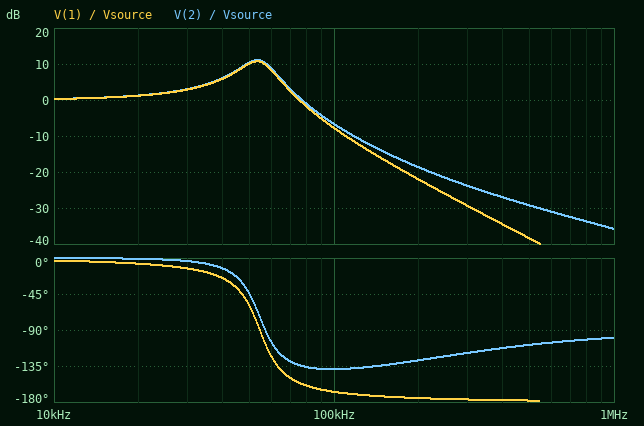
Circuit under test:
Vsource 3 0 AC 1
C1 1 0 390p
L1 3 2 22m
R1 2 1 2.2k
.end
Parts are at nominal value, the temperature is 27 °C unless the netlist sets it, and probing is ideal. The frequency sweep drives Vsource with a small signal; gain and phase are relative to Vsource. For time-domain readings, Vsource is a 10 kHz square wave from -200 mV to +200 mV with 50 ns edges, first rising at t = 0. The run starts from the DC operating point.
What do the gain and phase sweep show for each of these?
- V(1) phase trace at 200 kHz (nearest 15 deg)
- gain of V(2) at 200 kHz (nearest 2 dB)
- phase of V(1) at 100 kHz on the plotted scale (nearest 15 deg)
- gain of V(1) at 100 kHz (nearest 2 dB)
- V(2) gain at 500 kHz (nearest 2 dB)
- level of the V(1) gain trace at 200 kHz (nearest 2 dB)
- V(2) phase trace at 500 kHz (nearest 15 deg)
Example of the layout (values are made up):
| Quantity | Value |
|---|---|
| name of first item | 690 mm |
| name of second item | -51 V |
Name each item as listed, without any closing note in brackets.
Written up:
| Quantity | Value |
|---|---|
| V(1) phase trace at 200 kHz | -180 deg |
| gain of V(2) at 200 kHz | -18 dB |
| phase of V(1) at 100 kHz on the plotted scale | -165 deg |
| gain of V(1) at 100 kHz | -8 dB |
| V(2) gain at 500 kHz | -30 dB |
| level of the V(1) gain trace at 200 kHz | -22 dB |
| V(2) phase trace at 500 kHz | -105 deg |
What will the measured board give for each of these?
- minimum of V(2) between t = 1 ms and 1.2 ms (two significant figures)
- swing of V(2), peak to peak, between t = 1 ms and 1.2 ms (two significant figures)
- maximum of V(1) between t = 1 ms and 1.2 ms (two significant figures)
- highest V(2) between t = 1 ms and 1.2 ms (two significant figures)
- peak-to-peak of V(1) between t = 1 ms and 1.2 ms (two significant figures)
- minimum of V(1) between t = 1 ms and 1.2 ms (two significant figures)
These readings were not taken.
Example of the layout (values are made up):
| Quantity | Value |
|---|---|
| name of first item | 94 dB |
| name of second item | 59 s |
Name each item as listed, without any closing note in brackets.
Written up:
| Quantity | Value |
|---|---|
| minimum of V(2) between t = 1 ms and 1.2 ms | -470 mV |
| swing of V(2), peak to peak, between t = 1 ms and 1.2 ms | 950 mV |
| maximum of V(1) between t = 1 ms and 1.2 ms | 460 mV |
| highest V(2) between t = 1 ms and 1.2 ms | 470 mV |
| peak-to-peak of V(1) between t = 1 ms and 1.2 ms | 920 mV |
| minimum of V(1) between t = 1 ms and 1.2 ms | -460 mV |
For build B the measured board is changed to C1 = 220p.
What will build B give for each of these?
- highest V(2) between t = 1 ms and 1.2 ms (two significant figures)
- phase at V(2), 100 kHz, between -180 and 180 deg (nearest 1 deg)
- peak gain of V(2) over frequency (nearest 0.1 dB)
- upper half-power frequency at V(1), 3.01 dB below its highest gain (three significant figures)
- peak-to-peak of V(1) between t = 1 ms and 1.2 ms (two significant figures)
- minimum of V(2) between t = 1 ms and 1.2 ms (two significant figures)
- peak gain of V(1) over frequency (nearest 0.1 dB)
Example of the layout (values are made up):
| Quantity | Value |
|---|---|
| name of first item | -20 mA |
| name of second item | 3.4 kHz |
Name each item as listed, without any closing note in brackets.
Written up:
| Quantity | Value |
|---|---|
| highest V(2) between t = 1 ms and 1.2 ms | 510 mV |
| phase at V(2), 100 kHz, between -180 and 180 deg | -145 deg |
| peak gain of V(2) over frequency | 13.4 dB |
| upper half-power frequency at V(1), 3.01 dB below its highest gain | 79.1 kHz |
| peak-to-peak of V(1) between t = 1 ms and 1.2 ms | 1.0 V |
| minimum of V(2) between t = 1 ms and 1.2 ms | -510 mV |
| peak gain of V(1) over frequency | 13.2 dB |
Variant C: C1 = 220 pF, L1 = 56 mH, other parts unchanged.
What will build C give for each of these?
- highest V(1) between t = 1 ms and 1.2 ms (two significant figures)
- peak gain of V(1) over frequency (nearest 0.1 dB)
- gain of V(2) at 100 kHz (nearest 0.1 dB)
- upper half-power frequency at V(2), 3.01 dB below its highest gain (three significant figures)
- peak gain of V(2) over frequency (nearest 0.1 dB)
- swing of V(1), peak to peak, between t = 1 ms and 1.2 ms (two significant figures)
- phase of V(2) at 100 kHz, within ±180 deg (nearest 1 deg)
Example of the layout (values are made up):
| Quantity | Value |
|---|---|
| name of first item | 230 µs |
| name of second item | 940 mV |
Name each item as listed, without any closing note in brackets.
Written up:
| Quantity | Value |
|---|---|
| highest V(1) between t = 1 ms and 1.2 ms | 500 mV |
| peak gain of V(1) over frequency | 17.2 dB |
| gain of V(2) at 100 kHz | -11.4 dB |
| upper half-power frequency at V(2), 3.01 dB below its highest gain | 48.2 kHz |
| peak gain of V(2) over frequency | 17.3 dB |
| swing of V(1), peak to peak, between t = 1 ms and 1.2 ms | 1.0 V |
| phase of V(2) at 100 kHz, within ±180 deg | -159 deg |
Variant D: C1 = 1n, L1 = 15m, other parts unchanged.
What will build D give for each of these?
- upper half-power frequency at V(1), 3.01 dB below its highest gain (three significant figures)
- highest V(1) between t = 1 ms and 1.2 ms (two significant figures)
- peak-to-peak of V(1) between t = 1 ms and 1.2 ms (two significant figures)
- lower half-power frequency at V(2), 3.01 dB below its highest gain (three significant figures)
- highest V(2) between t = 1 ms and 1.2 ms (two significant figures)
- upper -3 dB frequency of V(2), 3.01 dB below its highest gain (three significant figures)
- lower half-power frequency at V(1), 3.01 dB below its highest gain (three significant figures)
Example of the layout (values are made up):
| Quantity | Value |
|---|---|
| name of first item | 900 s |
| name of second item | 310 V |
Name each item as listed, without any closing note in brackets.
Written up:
| Quantity | Value |
|---|---|
| upper half-power frequency at V(1), 3.01 dB below its highest gain | 48.3 kHz |
| highest V(1) between t = 1 ms and 1.2 ms | 350 mV |
| peak-to-peak of V(1) between t = 1 ms and 1.2 ms | 710 mV |
| lower half-power frequency at V(2), 3.01 dB below its highest gain | 24.9 kHz |
| highest V(2) between t = 1 ms and 1.2 ms | 380 mV |
| upper -3 dB frequency of V(2), 3.01 dB below its highest gain | 49.7 kHz |
| lower half-power frequency at V(1), 3.01 dB below its highest gain | 22.3 kHz |
